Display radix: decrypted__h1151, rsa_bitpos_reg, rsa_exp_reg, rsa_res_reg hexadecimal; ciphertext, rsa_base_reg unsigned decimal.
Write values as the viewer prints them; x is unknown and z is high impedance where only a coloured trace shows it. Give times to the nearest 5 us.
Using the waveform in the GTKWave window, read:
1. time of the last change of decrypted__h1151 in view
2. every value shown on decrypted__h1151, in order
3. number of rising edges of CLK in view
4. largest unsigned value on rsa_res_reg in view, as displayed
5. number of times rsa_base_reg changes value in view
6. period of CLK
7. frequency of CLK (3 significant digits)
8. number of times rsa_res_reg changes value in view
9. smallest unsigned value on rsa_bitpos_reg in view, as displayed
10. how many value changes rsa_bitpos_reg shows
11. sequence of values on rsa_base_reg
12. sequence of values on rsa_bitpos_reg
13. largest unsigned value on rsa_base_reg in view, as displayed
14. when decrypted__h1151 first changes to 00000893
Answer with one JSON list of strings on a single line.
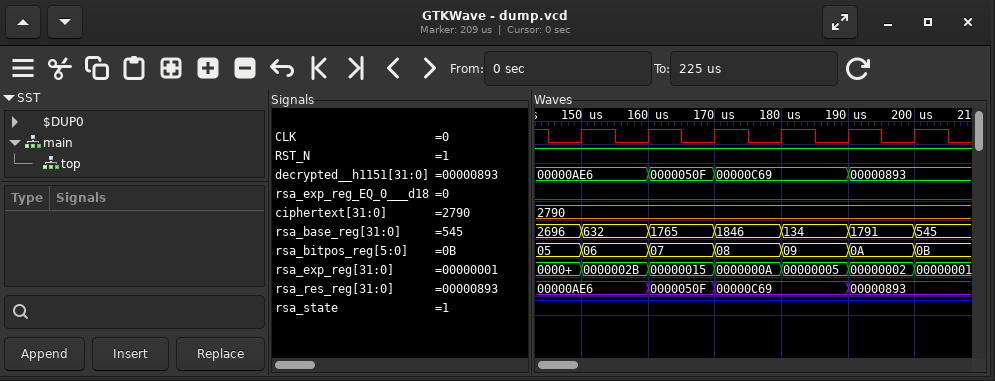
["190 us", "00000AE6, 0000050F, 00000C69, 00000893", "6", "00000C69", "6", "10 us", "100 kHz", "3", "05", "6", "2696, 632, 1765, 1846, 134, 1791, 545", "05, 06, 07, 08, 09, 0A, 0B", "2696", "190 us"]
